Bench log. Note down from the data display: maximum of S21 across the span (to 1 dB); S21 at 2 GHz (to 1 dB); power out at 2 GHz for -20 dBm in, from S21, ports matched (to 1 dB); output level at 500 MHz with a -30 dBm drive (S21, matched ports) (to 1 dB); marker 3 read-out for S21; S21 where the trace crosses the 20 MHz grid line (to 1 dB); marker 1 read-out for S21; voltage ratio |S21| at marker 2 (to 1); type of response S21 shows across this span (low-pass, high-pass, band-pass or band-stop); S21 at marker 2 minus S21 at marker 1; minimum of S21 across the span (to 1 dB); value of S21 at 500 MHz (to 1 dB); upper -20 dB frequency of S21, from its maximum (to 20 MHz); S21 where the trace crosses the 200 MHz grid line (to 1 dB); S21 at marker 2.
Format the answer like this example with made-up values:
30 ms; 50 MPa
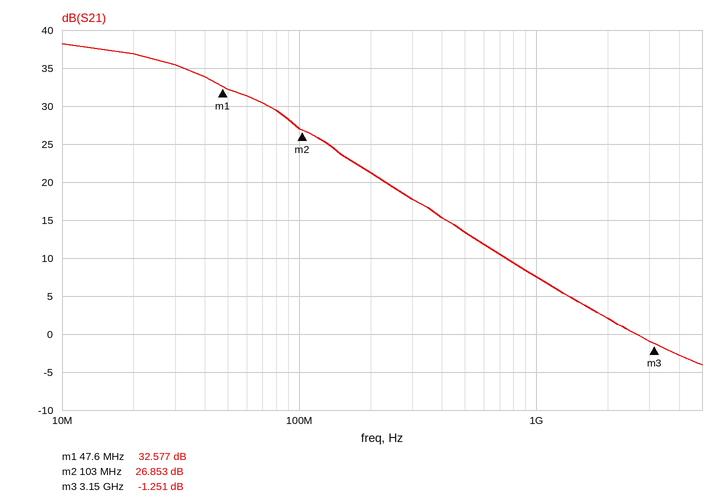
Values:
38 dB; 2 dB; -18 dBm; -17 dBm; -1.251 dB; 37 dB; 32.577 dB; 22; low-pass; -5.724 dB; -4 dB; 13 dB; 280 MHz; 21 dB; 26.853 dB
